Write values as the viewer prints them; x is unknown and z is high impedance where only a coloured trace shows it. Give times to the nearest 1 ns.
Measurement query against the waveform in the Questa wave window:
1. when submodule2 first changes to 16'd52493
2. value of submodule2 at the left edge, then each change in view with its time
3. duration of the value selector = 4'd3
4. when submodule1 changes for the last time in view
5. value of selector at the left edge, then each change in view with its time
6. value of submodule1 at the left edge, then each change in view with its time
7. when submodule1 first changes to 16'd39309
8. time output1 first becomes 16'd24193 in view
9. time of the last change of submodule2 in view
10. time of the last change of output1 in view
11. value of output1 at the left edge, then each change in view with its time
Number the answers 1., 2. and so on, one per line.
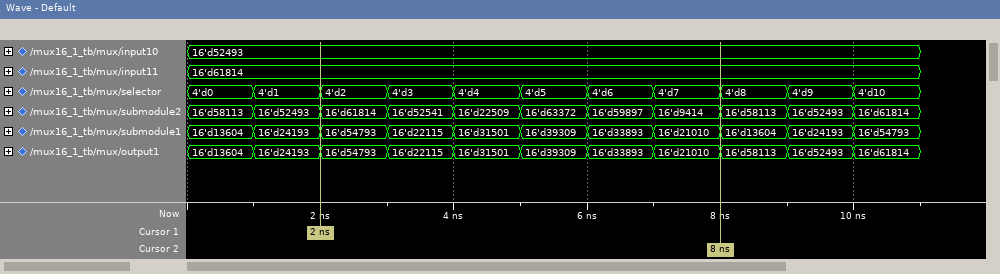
1. 1 ns
2. 16'd58113, 16'd52493 at 1 ns, 16'd61814 at 2 ns, 16'd52541 at 3 ns, 16'd22509 at 4 ns, 16'd63372 at 5 ns, 16'd59897 at 6 ns, 16'd9414 at 7 ns, 16'd58113 at 8 ns, 16'd52493 at 9 ns, 16'd61814 at 10 ns
3. 1 ns
4. 10 ns
5. 4'd0, 4'd1 at 1 ns, 4'd2 at 2 ns, 4'd3 at 3 ns, 4'd4 at 4 ns, 4'd5 at 5 ns, 4'd6 at 6 ns, 4'd7 at 7 ns, 4'd8 at 8 ns, 4'd9 at 9 ns, 4'd10 at 10 ns
6. 16'd13604, 16'd24193 at 1 ns, 16'd54793 at 2 ns, 16'd22115 at 3 ns, 16'd31501 at 4 ns, 16'd39309 at 5 ns, 16'd33893 at 6 ns, 16'd21010 at 7 ns, 16'd13604 at 8 ns, 16'd24193 at 9 ns, 16'd54793 at 10 ns
7. 5 ns
8. 1 ns
9. 10 ns
10. 10 ns
11. 16'd13604, 16'd24193 at 1 ns, 16'd54793 at 2 ns, 16'd22115 at 3 ns, 16'd31501 at 4 ns, 16'd39309 at 5 ns, 16'd33893 at 6 ns, 16'd21010 at 7 ns, 16'd58113 at 8 ns, 16'd52493 at 9 ns, 16'd61814 at 10 ns
